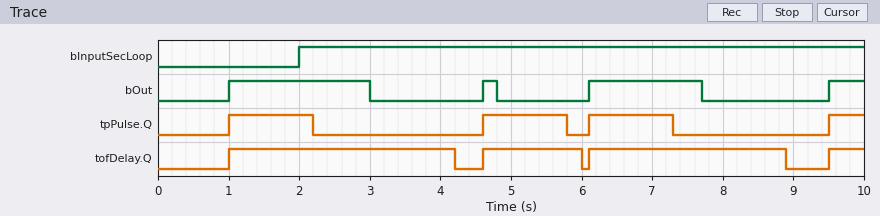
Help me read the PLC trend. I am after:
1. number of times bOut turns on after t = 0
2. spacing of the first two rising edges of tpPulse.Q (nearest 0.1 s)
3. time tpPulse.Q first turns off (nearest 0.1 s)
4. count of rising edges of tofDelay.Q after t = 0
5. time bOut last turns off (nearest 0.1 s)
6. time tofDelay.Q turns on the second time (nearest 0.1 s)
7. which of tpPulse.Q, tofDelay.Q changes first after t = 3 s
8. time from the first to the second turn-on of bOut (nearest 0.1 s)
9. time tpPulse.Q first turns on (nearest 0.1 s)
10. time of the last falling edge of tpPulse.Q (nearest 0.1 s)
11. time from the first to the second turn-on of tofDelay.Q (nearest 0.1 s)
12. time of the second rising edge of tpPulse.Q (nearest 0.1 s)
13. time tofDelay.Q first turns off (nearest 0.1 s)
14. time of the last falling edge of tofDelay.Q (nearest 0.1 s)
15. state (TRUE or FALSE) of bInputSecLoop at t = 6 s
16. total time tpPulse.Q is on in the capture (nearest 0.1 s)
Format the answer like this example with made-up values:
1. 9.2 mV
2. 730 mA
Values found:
1. 4
2. 3.6 s
3. 2.2 s
4. 4
5. 7.7 s
6. 4.6 s
7. tofDelay.Q
8. 3.6 s
9. 1.0 s
10. 7.3 s
11. 3.6 s
12. 4.6 s
13. 4.2 s
14. 8.9 s
15. TRUE
16. 4.1 s
